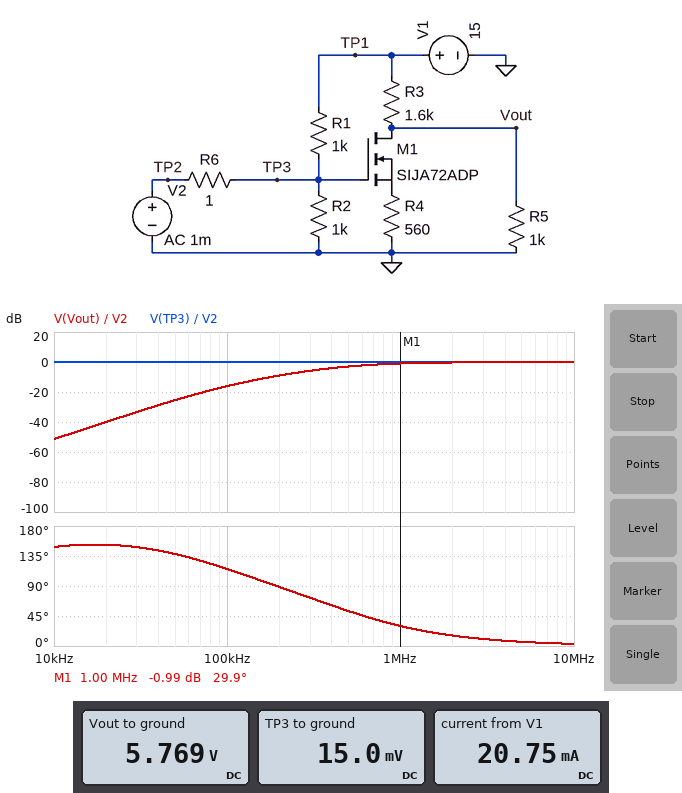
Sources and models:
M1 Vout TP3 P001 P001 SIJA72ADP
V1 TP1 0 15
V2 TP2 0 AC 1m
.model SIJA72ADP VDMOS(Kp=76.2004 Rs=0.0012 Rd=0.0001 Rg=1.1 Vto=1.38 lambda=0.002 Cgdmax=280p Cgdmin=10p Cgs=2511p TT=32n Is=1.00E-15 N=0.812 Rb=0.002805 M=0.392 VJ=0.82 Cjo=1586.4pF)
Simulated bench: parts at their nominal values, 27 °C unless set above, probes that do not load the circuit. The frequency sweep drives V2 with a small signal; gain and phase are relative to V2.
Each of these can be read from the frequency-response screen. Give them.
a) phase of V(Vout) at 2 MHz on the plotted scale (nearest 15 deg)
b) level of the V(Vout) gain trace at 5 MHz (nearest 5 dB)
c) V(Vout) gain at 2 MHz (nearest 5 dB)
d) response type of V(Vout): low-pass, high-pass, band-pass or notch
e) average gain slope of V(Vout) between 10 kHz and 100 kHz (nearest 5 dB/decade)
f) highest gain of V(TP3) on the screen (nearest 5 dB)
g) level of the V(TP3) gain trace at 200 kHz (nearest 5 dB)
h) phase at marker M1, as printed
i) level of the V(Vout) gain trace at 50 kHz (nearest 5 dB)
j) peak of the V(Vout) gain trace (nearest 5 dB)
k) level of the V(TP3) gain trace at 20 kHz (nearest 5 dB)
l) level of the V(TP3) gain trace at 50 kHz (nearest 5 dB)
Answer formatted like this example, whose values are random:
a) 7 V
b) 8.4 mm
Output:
a) 15 deg
b) 0 dB
c) 0 dB
d) high-pass
e) 35 dB/decade
f) 0 dB
g) 0 dB
h) 29.9 deg
i) -25 dB
j) 0 dB
k) 0 dB
l) 0 dB
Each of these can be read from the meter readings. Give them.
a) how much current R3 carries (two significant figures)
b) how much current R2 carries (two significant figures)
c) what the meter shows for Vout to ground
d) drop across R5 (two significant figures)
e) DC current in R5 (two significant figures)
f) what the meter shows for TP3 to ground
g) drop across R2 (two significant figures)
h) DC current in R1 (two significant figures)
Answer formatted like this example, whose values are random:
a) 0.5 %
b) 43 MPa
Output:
a) 5.8 mA
b) 15 µA
c) 5.769 V
d) 5.8 V
e) 5.8 mA
f) 15.0 mV
g) 15 mV
h) 15 mA
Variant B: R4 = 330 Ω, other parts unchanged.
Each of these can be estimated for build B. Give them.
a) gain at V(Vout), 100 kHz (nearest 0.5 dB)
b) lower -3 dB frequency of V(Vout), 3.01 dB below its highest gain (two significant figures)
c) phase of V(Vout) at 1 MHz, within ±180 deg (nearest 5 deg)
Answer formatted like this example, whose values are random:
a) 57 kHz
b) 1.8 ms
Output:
a) -18.5 dB
b) 530 kHz
c) 35 deg
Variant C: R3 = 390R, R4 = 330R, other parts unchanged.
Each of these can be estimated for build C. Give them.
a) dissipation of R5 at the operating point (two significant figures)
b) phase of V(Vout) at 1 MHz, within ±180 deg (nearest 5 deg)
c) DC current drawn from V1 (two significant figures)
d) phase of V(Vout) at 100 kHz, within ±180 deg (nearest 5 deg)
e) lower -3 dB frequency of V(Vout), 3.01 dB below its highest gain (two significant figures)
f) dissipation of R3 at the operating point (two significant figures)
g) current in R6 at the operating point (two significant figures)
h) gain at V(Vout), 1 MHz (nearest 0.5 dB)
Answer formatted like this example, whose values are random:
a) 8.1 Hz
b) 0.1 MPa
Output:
a) 120 mW
b) 60 deg
c) 26 mA
d) 140 deg
e) 1.2 MHz
f) 45 mW
g) 15 mA
h) -4.0 dB
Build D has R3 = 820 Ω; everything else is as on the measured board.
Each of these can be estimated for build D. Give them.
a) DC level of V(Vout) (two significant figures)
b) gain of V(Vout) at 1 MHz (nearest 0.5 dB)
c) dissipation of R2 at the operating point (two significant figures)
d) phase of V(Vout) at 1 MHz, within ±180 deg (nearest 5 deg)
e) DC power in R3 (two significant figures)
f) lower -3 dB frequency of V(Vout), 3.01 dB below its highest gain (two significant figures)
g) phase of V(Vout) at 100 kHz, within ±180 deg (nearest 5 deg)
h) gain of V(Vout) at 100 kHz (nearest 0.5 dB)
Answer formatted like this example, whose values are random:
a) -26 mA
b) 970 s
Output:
a) 8.2 V
b) -2.0 dB
c) 220 nW
d) 40 deg
e) 56 mW
f) 710 kHz
g) 120 deg
h) -19.5 dB
